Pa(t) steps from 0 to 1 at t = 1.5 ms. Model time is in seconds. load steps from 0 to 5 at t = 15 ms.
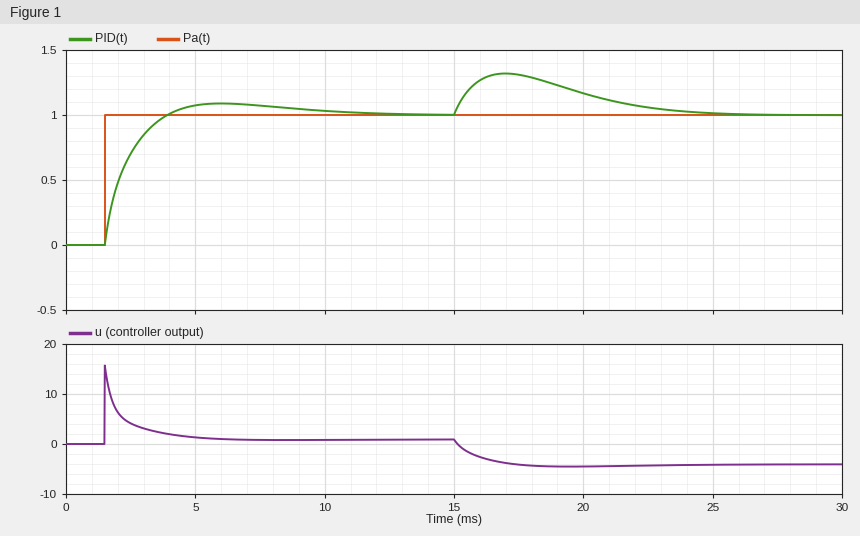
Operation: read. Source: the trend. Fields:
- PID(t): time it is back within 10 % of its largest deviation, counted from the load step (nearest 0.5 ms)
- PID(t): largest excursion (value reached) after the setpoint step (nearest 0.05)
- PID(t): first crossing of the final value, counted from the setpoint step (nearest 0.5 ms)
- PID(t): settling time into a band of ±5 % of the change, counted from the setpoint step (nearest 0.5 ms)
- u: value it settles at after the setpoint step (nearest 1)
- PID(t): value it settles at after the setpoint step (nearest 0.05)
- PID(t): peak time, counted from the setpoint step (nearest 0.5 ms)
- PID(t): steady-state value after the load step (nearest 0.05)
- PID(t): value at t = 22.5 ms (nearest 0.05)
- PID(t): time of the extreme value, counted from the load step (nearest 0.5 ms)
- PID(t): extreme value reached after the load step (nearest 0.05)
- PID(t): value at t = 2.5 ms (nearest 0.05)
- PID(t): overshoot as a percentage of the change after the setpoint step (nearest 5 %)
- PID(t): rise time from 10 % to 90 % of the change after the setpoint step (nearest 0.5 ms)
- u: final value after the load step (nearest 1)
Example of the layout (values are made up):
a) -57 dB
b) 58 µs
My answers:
a) 8.5 ms
b) 1.10
c) 2.5 ms
d) 7.5 ms
e) 1
f) 1.00
g) 4.5 ms
h) 1.00
i) 1.05
j) 2.0 ms
k) 1.30
l) 0.70
m) 10 %
n) 1.5 ms
o) -4
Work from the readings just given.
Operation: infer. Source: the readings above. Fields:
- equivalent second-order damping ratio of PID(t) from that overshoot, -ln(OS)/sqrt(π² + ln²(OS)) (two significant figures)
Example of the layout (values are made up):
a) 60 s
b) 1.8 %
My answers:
a) 0.59
